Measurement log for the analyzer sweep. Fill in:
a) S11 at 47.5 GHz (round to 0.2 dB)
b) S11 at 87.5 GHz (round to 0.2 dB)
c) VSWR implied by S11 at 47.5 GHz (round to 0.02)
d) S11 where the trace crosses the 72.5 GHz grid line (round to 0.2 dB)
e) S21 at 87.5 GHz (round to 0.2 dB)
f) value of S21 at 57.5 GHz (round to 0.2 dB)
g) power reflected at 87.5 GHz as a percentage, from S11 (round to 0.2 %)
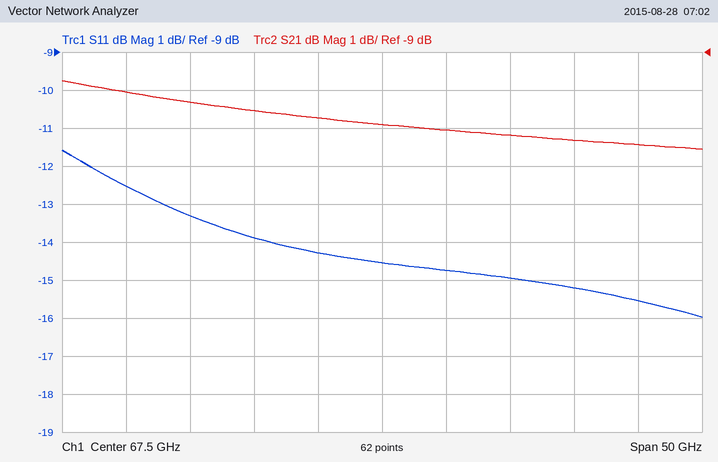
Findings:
-12.6 dB
-15.6 dB
1.62
-14.8 dB
-11.4 dB
-10.6 dB
2.8 %
